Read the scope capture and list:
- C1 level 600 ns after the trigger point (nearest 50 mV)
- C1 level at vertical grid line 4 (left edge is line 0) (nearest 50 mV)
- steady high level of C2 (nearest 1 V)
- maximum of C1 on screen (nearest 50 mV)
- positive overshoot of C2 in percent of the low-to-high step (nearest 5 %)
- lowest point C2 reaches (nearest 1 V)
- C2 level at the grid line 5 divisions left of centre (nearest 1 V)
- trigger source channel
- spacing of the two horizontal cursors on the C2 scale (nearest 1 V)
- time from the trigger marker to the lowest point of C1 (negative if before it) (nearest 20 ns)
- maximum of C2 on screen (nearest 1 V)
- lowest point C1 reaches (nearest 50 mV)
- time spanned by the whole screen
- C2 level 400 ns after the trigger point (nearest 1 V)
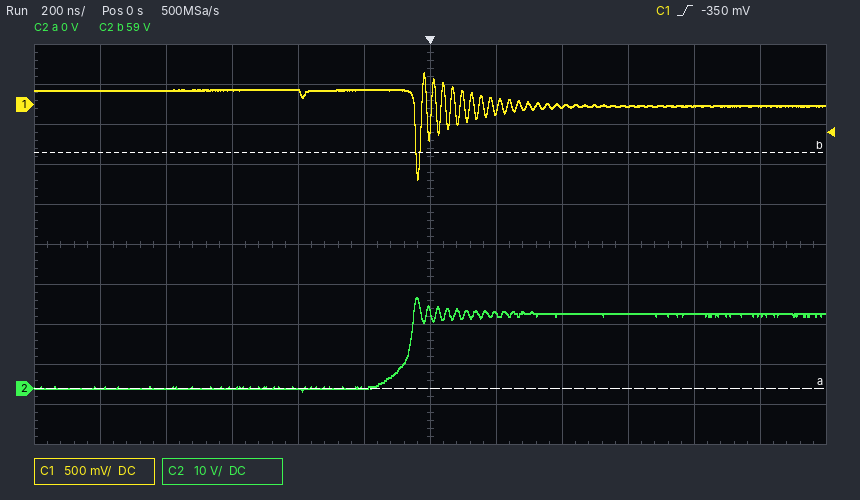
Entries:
0 mV
150 mV
19 V
400 mV
20 %
-1 V
0 V
C1
59 V
-40 ns
23 V
-950 mV
2.4 µs
19 V
